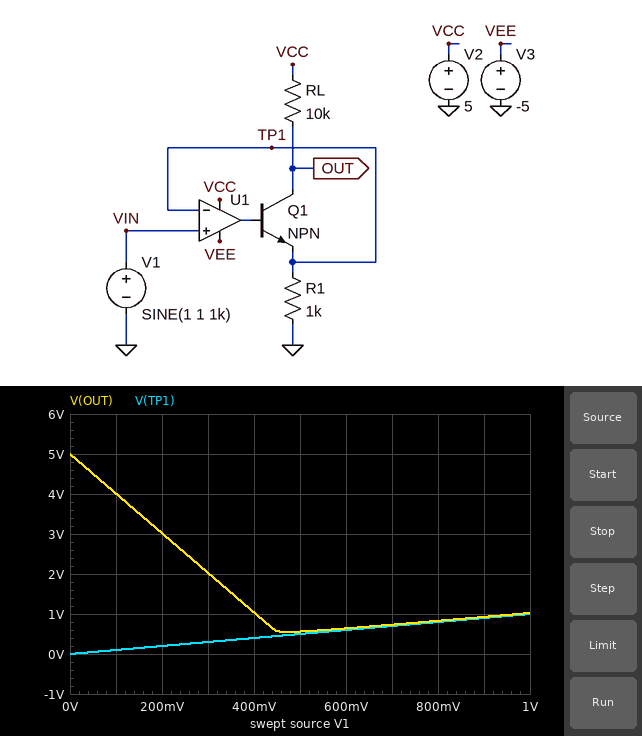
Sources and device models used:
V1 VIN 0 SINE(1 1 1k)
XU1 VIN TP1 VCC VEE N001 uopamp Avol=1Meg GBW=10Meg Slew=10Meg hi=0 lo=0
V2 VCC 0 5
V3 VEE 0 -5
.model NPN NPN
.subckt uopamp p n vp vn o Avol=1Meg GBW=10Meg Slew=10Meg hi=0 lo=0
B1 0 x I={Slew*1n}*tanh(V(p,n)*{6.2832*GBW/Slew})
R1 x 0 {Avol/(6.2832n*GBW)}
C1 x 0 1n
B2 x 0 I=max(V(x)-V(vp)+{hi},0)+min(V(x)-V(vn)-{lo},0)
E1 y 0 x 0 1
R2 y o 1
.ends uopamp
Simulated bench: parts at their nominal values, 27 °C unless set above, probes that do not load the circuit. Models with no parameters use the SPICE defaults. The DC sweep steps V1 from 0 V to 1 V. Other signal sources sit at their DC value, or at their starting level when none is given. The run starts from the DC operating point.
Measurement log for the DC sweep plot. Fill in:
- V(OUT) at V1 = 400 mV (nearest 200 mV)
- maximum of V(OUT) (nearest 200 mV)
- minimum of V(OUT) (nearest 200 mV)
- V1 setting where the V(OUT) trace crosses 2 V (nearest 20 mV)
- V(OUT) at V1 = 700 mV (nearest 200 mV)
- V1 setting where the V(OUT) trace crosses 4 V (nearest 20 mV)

1.0 V
5.0 V
600 mV
300 mV
800 mV
100 mV
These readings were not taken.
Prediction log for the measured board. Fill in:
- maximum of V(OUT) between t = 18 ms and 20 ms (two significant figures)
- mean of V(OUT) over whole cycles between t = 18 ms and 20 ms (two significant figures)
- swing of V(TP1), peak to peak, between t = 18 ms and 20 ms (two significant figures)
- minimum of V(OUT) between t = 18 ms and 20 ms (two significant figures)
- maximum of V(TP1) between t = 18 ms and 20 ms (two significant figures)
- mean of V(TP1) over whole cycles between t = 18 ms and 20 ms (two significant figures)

5.0 V
2.1 V
2.0 V
550 mV
2.0 V
1.0 V
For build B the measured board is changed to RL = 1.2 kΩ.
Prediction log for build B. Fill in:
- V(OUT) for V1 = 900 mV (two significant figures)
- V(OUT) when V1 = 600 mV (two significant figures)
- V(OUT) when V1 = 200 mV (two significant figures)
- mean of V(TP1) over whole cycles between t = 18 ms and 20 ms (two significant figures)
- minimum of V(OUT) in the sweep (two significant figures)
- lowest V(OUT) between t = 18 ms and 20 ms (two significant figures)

3.9 V
4.3 V
4.8 V
1.0 V
3.8 V
2.6 V
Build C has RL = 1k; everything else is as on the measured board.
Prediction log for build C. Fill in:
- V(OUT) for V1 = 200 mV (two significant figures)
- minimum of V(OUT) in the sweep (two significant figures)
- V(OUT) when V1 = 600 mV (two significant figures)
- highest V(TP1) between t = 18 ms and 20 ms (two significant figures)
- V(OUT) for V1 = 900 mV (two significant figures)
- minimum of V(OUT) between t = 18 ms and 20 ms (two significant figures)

4.8 V
4.0 V
4.4 V
2.0 V
4.1 V
3.0 V
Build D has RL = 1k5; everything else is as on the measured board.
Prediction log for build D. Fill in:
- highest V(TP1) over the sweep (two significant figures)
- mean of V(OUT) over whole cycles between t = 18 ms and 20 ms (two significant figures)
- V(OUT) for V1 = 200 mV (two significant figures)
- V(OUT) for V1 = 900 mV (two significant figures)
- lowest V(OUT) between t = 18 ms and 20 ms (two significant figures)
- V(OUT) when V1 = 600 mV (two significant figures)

1.0 V
3.5 V
4.7 V
3.7 V
2.1 V
4.1 V
